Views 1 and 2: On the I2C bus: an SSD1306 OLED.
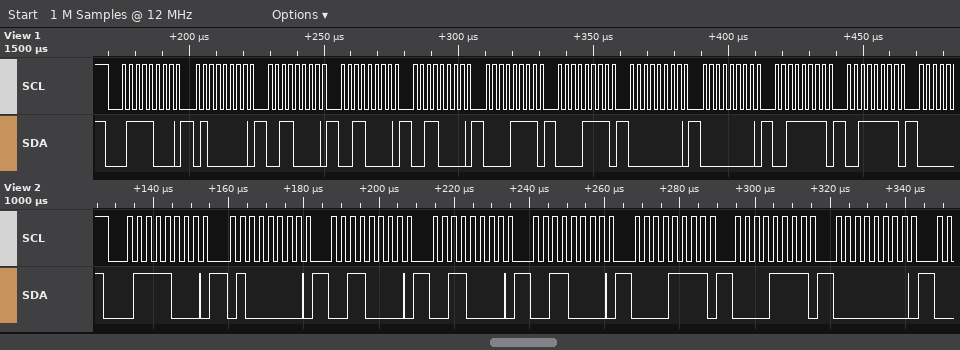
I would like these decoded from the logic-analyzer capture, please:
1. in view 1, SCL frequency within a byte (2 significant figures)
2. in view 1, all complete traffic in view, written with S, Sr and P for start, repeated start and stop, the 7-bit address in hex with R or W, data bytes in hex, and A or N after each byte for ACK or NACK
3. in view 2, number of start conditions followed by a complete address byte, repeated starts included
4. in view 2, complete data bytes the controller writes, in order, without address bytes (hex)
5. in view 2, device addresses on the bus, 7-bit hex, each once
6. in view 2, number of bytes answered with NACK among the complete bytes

400 kHz
S 3CW A 40 A 30 A 30 A 30 A 0F A 0F A 00 A 00 A 3F A 3F A
1
40 30 30 30 0F 0F 00
0x3C
0
